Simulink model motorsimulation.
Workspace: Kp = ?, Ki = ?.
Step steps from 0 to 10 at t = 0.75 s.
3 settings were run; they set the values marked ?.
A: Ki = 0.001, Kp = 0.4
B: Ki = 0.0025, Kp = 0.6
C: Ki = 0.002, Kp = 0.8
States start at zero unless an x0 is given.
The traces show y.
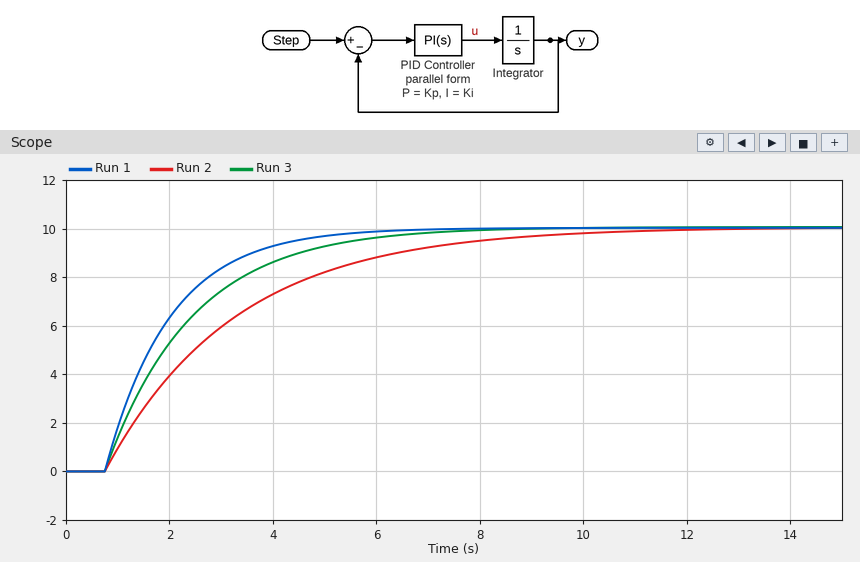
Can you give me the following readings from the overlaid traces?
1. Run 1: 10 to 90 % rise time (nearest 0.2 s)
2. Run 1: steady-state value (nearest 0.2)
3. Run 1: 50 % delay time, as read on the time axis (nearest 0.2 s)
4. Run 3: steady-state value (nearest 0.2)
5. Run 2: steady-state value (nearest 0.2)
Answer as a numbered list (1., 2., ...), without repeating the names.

1. 2.8 s
2. 10.0
3. 1.6 s
4. 10.0
5. 10.0
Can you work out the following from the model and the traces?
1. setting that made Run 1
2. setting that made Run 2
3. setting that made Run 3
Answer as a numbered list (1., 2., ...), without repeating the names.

1. C
2. A
3. B
